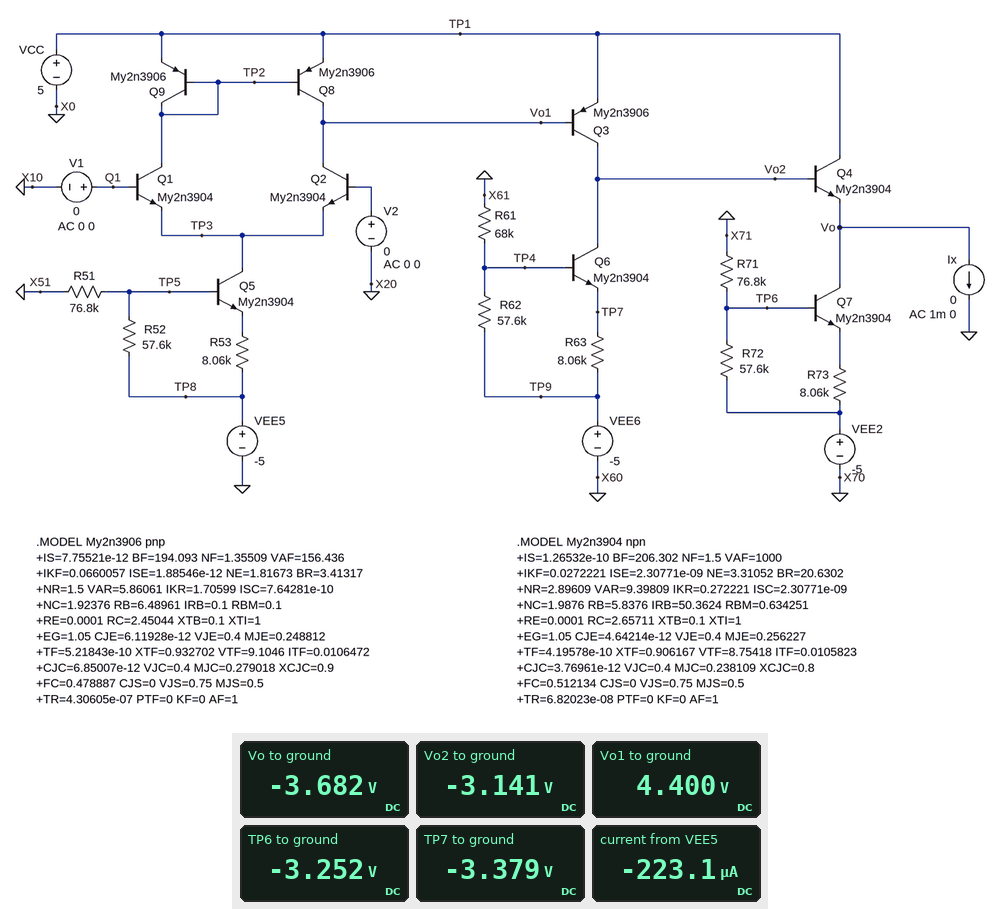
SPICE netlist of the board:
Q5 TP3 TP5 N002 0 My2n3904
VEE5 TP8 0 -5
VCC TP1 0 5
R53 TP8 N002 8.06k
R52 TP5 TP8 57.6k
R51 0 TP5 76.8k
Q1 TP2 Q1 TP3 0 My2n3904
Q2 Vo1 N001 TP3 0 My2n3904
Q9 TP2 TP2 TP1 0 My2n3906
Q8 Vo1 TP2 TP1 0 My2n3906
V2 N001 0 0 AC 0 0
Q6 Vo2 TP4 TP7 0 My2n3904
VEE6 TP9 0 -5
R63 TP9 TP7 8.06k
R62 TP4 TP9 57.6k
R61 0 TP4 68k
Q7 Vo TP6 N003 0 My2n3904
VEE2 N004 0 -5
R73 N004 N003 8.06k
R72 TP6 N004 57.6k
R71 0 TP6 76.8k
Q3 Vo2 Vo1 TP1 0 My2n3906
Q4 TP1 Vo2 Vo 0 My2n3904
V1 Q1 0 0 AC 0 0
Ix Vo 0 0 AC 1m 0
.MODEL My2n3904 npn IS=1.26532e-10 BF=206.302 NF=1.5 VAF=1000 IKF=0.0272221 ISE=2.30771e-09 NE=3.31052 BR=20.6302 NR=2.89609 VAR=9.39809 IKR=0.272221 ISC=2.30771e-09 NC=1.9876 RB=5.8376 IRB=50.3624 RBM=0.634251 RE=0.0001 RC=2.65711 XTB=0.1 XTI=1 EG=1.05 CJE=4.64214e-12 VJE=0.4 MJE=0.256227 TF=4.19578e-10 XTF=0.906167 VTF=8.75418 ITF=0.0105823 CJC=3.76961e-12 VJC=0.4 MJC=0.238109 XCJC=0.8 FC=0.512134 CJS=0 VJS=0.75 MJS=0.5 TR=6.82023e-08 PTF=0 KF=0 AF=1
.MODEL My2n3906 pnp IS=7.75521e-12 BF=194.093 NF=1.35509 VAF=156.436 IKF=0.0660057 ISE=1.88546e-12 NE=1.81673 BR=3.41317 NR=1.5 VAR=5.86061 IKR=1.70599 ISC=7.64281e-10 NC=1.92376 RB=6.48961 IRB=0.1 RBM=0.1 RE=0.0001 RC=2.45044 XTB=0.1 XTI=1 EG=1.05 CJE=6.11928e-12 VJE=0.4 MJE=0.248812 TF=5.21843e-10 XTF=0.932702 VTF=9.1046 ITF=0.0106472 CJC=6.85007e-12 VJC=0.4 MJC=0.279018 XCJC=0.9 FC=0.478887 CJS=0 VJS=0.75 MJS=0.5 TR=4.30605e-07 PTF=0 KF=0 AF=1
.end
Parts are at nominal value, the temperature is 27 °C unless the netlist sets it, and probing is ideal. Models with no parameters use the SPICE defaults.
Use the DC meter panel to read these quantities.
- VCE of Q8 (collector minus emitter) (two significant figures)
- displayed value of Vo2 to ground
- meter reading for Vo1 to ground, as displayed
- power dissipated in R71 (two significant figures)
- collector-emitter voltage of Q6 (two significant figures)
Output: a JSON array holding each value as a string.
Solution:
["-600 mV", "-3.141 V", "4.400 V", "140 µW", "240 mV"]
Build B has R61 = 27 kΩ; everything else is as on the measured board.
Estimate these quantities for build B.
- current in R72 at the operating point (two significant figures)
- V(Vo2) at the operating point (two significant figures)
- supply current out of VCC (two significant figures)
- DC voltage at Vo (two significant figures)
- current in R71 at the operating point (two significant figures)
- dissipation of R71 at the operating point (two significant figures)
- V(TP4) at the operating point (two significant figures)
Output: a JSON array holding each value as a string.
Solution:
["33 µA", "-3.0 V", "540 µA", "-3.5 V", "41 µA", "130 µW", "-2.5 V"]
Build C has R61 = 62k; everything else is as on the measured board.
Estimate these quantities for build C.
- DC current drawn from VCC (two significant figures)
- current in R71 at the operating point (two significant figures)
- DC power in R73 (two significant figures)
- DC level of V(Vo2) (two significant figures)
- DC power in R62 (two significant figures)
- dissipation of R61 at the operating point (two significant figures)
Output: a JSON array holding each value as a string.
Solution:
["510 µA", "43 µA", "170 µW", "-3.2 V", "84 µW", "130 µW"]
